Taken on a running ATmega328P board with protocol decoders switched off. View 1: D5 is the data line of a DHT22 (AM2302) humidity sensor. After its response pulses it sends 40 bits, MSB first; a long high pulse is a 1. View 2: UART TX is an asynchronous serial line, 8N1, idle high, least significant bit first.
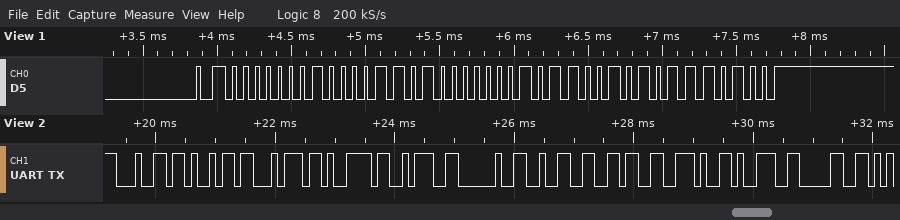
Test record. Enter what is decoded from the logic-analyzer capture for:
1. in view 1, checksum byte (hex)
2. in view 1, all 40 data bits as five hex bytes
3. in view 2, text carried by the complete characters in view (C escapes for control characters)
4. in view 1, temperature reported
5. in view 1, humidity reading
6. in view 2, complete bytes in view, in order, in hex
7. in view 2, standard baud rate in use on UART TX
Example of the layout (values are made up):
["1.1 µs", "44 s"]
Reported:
["0x74", "01 0D 01 65 74", "\"dity: 26.90\"", "35.7 °C", "26.9 %", "64 69 74 79 3A 20 32 36 2E 39 30", "9600 baud"]
